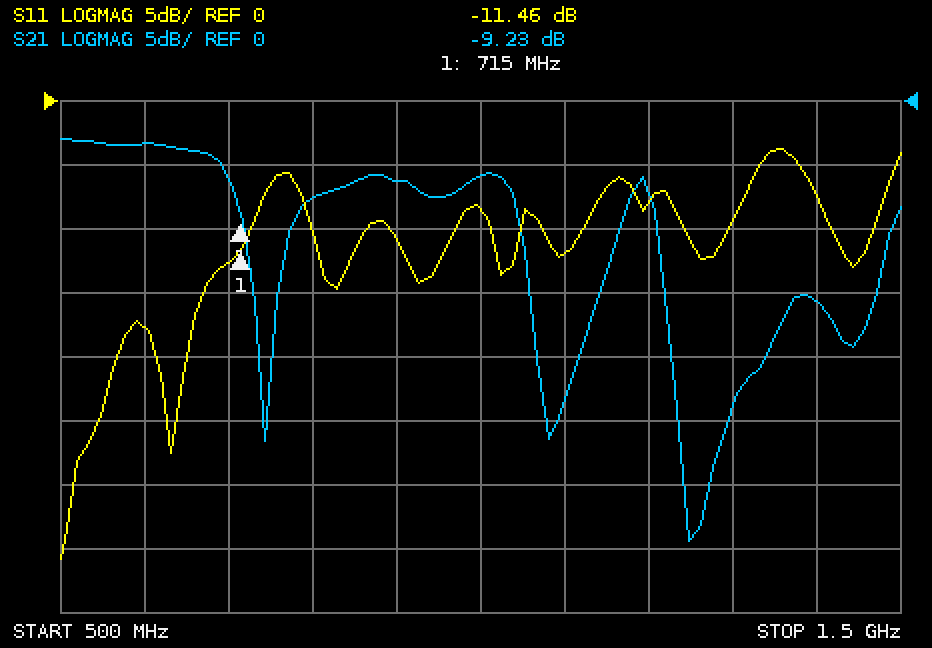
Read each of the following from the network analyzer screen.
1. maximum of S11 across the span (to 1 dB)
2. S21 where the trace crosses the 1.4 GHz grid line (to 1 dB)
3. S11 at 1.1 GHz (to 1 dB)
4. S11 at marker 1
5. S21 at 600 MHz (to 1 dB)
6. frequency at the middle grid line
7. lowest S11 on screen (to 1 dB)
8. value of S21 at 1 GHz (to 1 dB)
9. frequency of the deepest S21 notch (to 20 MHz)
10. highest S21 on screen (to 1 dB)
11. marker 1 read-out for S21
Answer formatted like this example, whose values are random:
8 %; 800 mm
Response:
-4 dB; -16 dB; -12 dB; -11.46 dB; -3 dB; 1 GHz; -36 dB; -6 dB; 1.24 GHz; -3 dB; -9.23 dB
